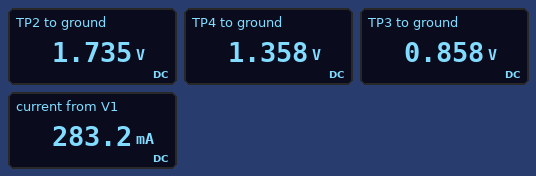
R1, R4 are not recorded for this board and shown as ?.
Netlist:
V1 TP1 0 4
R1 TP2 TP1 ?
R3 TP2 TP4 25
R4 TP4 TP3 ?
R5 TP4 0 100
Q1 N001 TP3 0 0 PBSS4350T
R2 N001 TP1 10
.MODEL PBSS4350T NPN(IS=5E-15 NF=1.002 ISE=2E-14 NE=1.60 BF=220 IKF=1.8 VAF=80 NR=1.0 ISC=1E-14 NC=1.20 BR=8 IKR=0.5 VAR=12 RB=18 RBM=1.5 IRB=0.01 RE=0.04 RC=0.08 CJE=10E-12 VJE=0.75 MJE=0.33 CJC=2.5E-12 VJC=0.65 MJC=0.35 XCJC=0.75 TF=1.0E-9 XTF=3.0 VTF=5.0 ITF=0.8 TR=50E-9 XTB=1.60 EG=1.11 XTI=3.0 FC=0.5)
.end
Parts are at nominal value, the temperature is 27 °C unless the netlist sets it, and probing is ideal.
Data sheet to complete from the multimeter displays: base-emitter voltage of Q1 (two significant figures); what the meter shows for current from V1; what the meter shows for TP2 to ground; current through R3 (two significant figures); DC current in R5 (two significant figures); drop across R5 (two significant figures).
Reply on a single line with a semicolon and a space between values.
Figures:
860 mV; 283.2 mA; 1.735 V; 15 mA; 14 mA; 1.4 V
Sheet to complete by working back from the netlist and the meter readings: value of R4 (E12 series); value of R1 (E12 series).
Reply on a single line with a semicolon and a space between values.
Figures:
330 Ω; 150 Ω
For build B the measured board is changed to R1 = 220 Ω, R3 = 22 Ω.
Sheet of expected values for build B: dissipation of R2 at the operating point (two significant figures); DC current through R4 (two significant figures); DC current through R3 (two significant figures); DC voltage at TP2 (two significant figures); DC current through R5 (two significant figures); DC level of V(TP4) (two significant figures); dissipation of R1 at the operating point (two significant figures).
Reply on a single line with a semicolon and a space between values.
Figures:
260 mW; 850 µA; 12 mA; 1.4 V; 11 mA; 1.1 V; 31 mW
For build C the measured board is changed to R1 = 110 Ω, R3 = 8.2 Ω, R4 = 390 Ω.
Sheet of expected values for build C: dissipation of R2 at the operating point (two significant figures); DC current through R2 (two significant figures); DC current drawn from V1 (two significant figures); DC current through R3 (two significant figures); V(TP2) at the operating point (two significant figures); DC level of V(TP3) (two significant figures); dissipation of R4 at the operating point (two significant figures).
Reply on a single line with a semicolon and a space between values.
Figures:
1.3 W; 360 mA; 380 mA; 19 mA; 1.9 V; 880 mV; 1.8 mW
